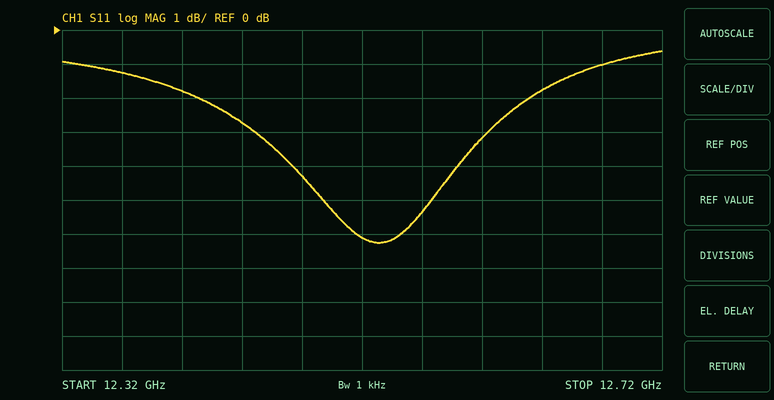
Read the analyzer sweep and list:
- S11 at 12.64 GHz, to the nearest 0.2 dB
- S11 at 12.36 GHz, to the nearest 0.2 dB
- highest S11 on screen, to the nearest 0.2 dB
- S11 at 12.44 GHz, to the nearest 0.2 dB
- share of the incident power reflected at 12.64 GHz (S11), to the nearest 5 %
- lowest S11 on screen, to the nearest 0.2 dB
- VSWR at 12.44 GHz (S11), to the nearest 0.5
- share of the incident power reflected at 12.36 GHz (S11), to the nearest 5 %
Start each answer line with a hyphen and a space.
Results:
- -1.8 dB
- -1.2 dB
- -0.6 dB
- -2.8 dB
- 65 %
- -6.2 dB
- 6.5
- 75 %
